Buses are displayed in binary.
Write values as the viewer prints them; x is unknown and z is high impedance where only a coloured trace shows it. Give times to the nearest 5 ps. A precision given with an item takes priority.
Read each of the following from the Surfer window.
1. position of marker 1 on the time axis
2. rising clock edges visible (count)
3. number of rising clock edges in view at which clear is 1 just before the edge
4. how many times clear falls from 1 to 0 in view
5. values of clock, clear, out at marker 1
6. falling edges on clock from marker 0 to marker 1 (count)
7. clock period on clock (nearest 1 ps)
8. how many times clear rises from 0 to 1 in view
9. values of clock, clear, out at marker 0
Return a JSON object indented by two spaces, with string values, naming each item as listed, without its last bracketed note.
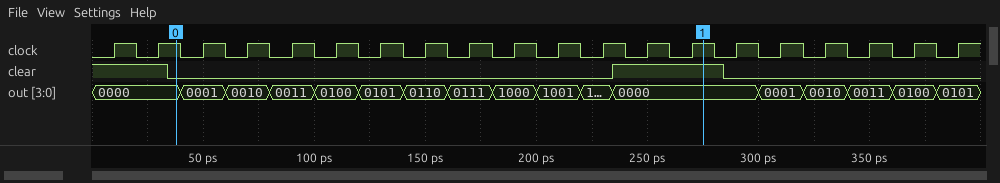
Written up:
{
  "position of marker 1 on the time axis": "275 ps",
  "rising clock edges visible": "20",
  "number of rising clock edges in view at which clear is 1 just before the edge": "4",
  "how many times clear falls from 1 to 0 in view": "2",
  "values of clock, clear, out at marker 1": "clock=1, clear=1, out=0000",
  "falling edges on clock from marker 0 to marker 1": "12",
  "clock period on clock": "20 ps",
  "how many times clear rises from 0 to 1 in view": "1",
  "values of clock, clear, out at marker 0": "clock=1, clear=0, out=0000"
}
